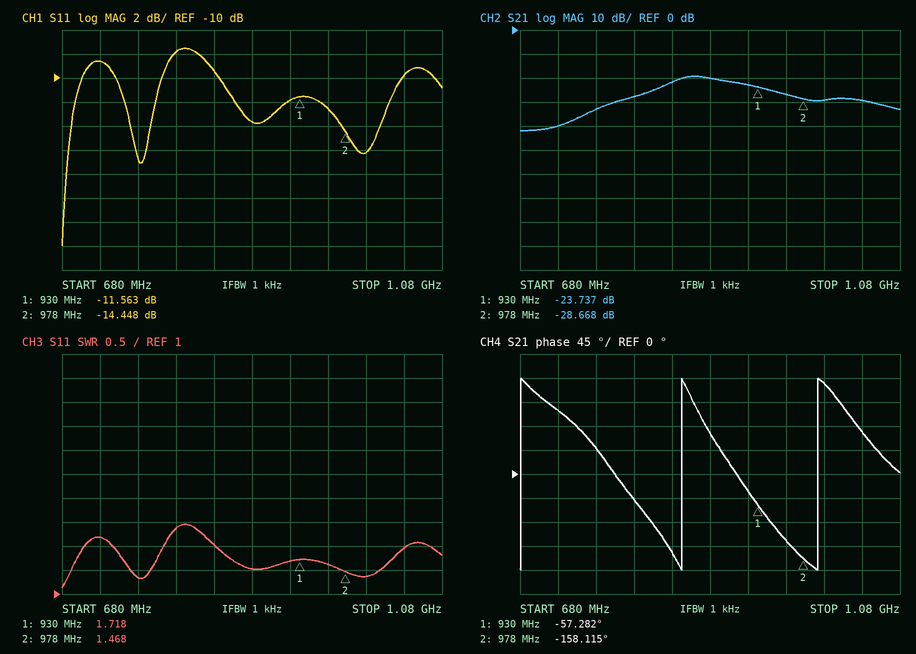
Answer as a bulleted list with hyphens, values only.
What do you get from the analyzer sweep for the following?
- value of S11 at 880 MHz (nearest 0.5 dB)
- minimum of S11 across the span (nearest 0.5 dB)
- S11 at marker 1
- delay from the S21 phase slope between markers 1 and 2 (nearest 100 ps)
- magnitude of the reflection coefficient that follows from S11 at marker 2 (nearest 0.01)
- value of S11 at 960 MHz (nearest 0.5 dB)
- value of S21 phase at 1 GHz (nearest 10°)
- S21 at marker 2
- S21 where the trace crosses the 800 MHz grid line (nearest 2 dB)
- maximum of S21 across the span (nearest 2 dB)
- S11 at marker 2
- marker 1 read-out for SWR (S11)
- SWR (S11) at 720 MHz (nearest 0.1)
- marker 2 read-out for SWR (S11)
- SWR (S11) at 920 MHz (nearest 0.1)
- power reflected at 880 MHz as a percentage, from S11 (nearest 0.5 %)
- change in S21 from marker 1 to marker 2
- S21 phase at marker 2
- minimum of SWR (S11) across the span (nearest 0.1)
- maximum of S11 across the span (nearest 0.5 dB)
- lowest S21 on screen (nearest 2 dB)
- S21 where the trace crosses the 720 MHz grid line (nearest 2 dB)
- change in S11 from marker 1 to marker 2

- -13.5 dB
- -24.0 dB
- -11.563 dB
- 5.8 ns
- 0.19
- -12.5 dB
- 170°
- -28.668 dB
- -28 dB
- -20 dB
- -14.448 dB
- 1.718
- 2.2
- 1.468
- 1.7
- 4.5 %
- -4.931 dB
- -158.115°
- 1.1
- -7.5 dB
- -42 dB
- -40 dB
- -2.885 dB
